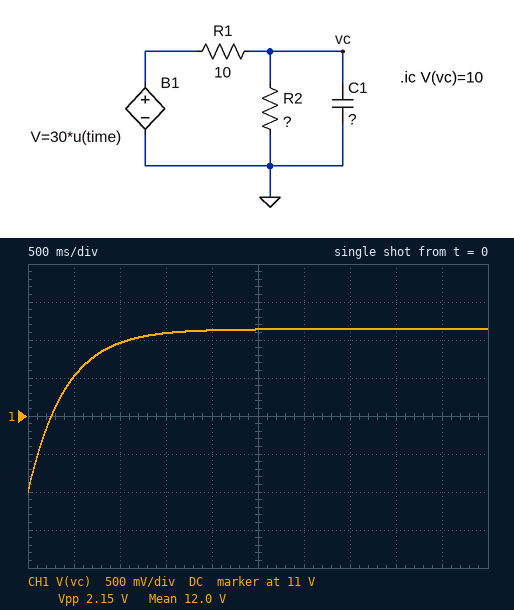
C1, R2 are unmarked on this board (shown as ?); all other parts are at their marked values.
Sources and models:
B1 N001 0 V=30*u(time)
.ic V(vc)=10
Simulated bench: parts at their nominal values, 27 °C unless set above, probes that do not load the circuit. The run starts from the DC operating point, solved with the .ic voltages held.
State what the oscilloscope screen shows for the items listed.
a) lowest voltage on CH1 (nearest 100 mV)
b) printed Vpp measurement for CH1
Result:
10.0 V
2.15 V
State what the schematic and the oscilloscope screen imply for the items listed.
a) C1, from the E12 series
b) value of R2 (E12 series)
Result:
100 mF
6.8 Ω
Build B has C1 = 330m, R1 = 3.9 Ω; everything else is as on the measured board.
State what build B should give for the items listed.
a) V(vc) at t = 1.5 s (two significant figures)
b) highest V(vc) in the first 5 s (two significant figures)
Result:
18 V
19 V
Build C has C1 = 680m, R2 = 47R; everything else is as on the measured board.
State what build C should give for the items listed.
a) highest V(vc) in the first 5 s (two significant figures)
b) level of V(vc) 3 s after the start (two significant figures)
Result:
19 V
16 V
